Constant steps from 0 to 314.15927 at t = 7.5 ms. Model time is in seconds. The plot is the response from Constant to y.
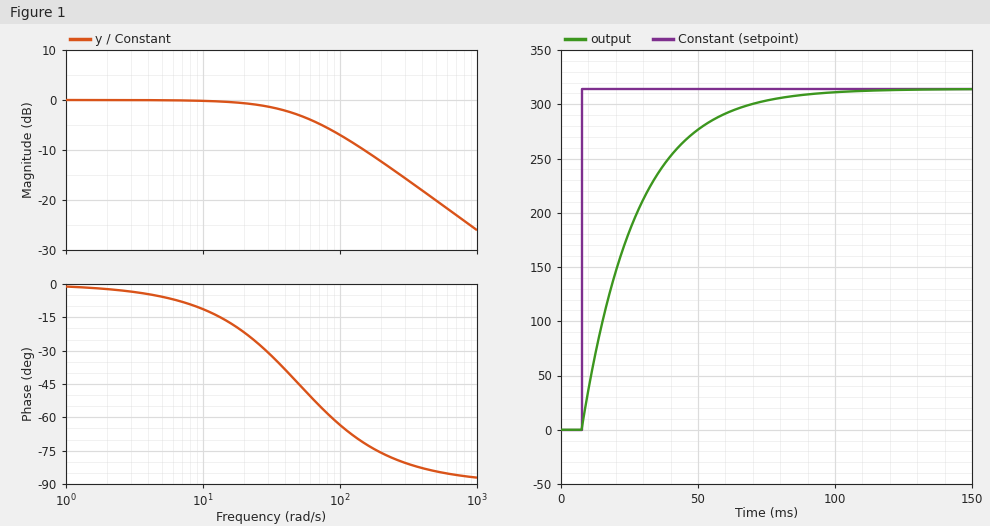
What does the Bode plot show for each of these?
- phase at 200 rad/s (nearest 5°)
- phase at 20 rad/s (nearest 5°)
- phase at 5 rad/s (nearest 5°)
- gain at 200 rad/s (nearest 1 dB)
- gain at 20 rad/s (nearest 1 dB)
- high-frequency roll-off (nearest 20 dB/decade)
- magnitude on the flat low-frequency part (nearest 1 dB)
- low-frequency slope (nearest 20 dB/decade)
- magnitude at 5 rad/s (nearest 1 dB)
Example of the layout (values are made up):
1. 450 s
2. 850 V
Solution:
1. -75°
2. -20°
3. -5°
4. -12 dB
5. -1 dB
6. -20 dB/decade
7. 0 dB
8. 0 dB/decade
9. 0 dB
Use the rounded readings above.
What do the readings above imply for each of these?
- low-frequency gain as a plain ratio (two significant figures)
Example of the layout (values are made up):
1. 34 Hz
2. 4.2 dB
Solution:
1. 1.0
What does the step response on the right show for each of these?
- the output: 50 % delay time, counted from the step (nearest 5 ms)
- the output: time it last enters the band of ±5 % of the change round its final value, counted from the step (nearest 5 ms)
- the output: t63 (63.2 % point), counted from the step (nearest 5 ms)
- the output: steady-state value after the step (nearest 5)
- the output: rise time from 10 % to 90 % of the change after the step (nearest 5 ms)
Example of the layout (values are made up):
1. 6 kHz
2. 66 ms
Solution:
1. 15 ms
2. 60 ms
3. 20 ms
4. 315
5. 45 ms
